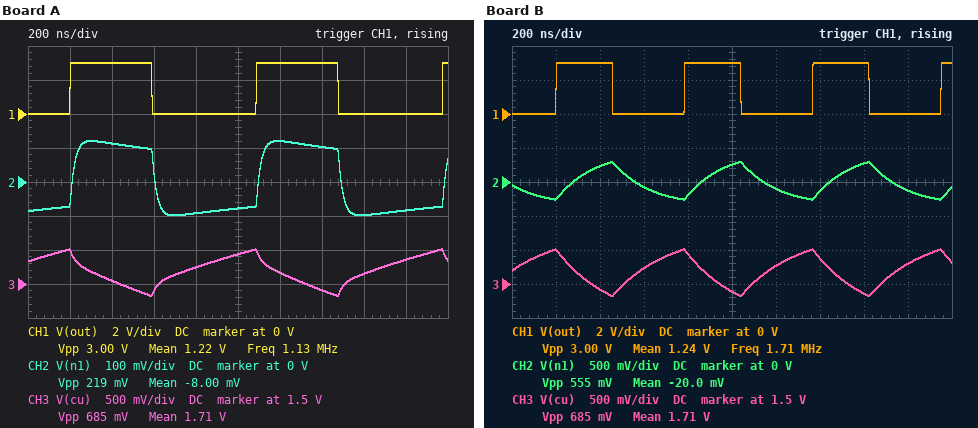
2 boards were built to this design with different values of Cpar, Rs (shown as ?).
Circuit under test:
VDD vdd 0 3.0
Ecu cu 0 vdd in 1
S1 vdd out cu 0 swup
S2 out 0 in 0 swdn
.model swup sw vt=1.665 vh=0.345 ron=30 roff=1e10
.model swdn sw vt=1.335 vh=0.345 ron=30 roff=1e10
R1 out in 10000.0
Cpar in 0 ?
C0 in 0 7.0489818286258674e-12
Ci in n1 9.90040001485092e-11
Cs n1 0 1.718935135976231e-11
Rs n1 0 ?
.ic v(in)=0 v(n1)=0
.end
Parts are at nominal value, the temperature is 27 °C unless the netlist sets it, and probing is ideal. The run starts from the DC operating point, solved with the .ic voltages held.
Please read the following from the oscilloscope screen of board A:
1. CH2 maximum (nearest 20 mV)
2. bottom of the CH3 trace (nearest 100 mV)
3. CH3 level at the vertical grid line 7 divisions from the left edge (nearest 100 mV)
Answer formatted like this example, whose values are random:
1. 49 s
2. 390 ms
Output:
1. 120 mV
2. 1.3 V
3. 1.4 V
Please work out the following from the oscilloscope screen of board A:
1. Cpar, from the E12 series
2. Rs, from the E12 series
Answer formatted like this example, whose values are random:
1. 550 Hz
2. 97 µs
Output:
1. 6.8 pF
2. 820 Ω
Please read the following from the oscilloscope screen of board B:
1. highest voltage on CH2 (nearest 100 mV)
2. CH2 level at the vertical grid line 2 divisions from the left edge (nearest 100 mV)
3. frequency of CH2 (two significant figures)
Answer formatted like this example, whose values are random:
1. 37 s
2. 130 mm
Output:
1. 300 mV
2. 200 mV
3. 1.7 MHz
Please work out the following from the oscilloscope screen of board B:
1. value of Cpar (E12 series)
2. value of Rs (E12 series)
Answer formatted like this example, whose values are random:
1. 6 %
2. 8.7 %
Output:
1. 33 pF
2. 5.6 kΩ
